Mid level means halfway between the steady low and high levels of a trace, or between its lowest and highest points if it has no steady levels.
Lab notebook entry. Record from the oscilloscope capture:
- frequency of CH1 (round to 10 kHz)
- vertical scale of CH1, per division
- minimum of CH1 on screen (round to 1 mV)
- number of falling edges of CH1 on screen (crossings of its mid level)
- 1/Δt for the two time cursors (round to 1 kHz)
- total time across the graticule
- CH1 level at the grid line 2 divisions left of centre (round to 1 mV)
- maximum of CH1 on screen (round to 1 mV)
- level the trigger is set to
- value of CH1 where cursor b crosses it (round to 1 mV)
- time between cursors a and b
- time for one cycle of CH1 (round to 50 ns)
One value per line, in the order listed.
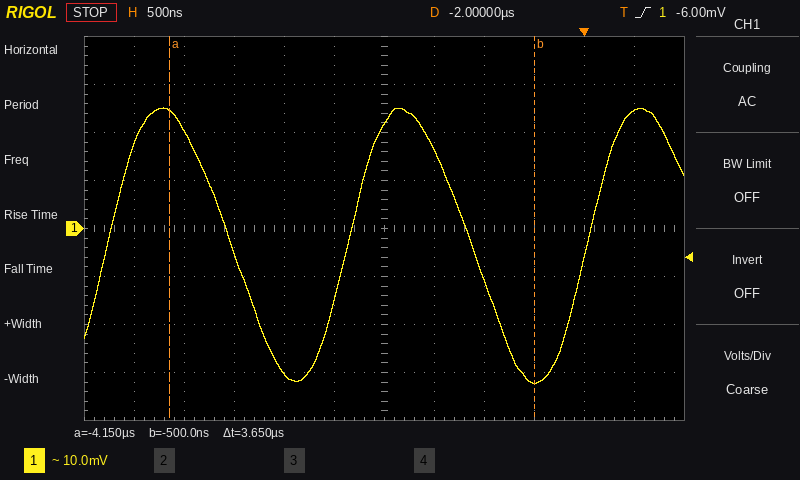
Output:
420 kHz
10 mV
-32 mV
2
274 kHz
6 µs
-30 mV
25 mV
-6.00 mV
-32 mV
3.65 µs
2.40 µs
